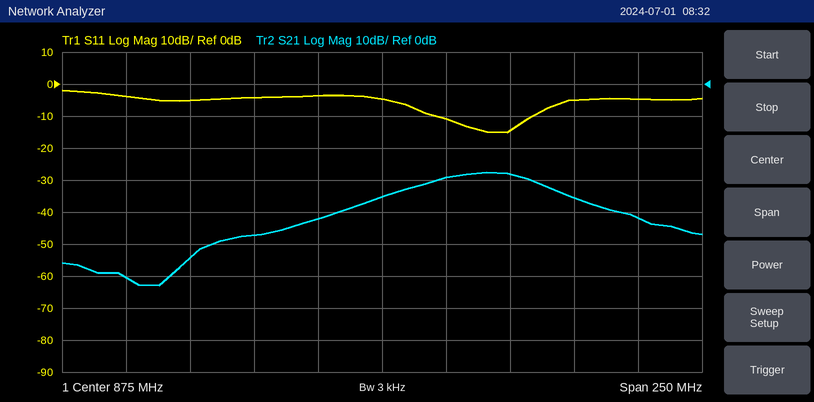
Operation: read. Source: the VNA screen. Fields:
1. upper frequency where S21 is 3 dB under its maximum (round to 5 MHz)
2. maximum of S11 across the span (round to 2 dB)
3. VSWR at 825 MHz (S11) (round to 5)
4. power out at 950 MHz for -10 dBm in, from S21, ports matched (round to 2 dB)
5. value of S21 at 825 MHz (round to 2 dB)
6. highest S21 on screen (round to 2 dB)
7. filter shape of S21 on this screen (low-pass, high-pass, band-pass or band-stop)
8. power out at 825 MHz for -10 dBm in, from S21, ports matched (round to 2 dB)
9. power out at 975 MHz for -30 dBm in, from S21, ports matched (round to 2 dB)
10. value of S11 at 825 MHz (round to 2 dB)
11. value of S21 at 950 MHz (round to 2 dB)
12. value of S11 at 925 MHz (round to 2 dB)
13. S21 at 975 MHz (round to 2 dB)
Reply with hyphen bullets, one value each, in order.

- 935 MHz
- -2 dB
- 5
- -46 dBm
- -48 dB
- -28 dB
- band-pass
- -58 dBm
- -72 dBm
- -4 dB
- -36 dB
- -14 dB
- -42 dB
